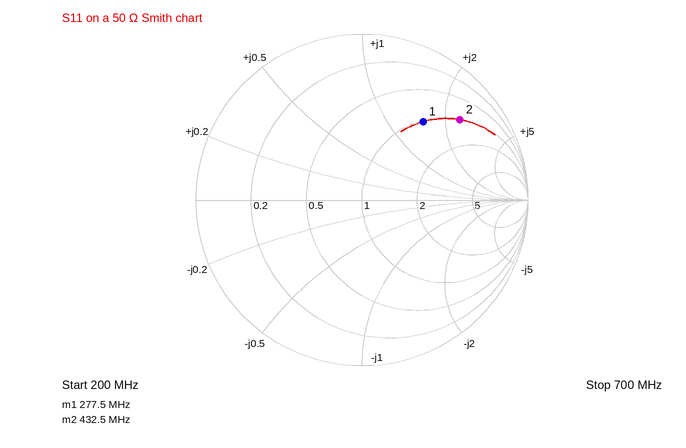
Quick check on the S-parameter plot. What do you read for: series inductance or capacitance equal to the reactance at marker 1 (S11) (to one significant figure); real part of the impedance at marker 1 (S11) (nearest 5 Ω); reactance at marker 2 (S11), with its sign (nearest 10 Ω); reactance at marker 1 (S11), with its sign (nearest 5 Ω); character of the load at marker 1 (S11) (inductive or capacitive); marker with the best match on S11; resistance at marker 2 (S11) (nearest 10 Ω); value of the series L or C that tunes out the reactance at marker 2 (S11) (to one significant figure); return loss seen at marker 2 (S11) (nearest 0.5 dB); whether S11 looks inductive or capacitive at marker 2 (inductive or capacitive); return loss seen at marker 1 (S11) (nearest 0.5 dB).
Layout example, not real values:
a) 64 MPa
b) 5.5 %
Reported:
a) 40 nH
b) 50 Ω
c) +120 Ω
d) +75 Ω
e) inductive
f) marker 1
g) 50 Ω
h) 3 pF
i) 2.5 dB
j) inductive
k) 4.5 dB
